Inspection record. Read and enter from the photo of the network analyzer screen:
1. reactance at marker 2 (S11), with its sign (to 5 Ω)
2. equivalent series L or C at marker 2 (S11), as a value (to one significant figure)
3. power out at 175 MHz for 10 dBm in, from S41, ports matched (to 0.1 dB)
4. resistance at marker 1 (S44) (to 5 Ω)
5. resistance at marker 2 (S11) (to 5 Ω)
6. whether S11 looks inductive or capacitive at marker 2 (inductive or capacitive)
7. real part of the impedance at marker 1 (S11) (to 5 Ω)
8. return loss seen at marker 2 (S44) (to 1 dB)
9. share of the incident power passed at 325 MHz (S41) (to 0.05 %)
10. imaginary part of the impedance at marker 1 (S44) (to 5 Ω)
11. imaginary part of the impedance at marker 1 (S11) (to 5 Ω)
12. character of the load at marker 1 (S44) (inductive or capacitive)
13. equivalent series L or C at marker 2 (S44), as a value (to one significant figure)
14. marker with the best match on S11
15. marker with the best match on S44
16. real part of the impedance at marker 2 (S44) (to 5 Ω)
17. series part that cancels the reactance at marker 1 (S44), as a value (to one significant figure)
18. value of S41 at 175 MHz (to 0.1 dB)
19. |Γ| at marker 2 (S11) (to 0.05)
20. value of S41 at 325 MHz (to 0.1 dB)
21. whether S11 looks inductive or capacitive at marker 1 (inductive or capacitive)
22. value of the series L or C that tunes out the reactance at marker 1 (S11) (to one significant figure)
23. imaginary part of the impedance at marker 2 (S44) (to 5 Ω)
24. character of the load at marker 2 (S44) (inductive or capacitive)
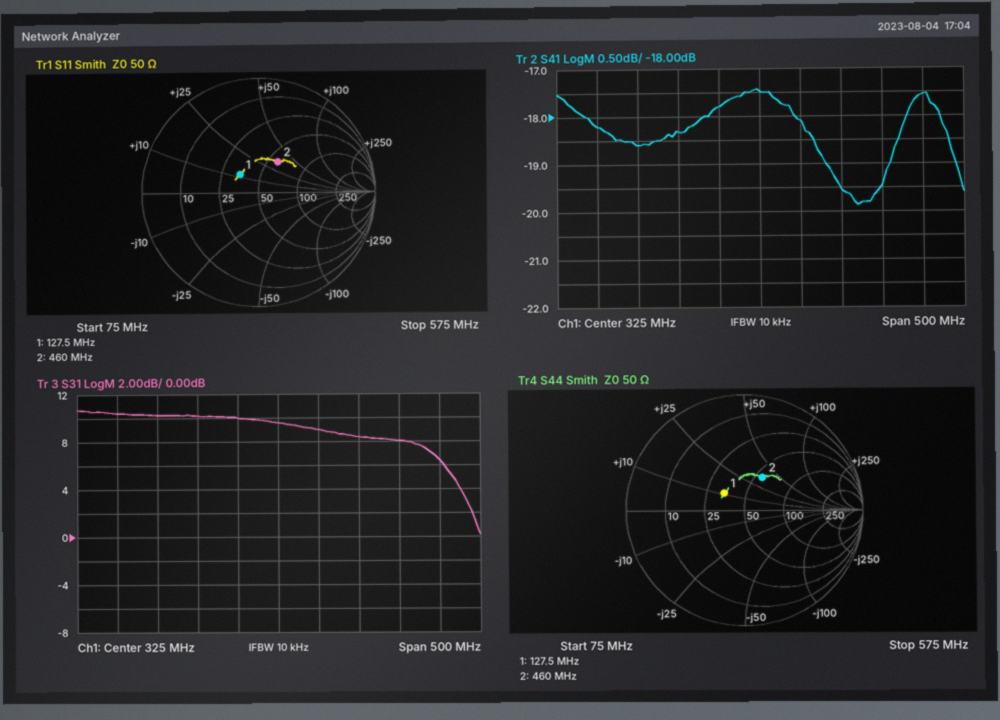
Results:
+35 Ω
10 nH
-8.6 dBm
35 Ω
60 Ω
inductive
35 Ω
10 dB
1.80 %
+10 Ω
+10 Ω
inductive
10 nH
marker 1
marker 1
55 Ω
100 pF
-18.6 dB
0.30
-17.5 dB
inductive
100 pF
+35 Ω
inductive
